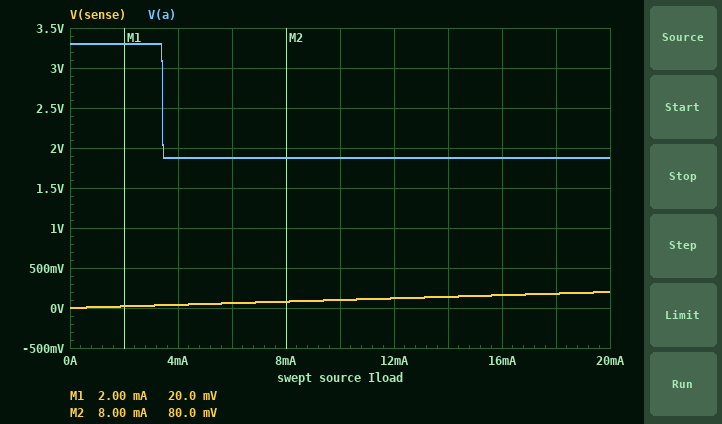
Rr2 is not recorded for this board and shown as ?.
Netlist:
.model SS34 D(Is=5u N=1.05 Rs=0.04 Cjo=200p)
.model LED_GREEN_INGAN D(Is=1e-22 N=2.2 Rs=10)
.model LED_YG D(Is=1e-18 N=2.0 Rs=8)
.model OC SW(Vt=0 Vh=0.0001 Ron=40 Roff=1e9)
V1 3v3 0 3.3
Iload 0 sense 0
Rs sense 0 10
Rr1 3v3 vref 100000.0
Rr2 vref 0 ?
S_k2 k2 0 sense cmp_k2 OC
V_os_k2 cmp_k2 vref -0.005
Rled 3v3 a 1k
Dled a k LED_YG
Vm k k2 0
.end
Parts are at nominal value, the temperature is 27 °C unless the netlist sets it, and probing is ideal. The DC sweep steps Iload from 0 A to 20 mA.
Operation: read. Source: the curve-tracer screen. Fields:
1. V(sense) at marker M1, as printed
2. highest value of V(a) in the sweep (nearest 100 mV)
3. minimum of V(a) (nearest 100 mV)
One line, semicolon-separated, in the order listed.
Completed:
20.0 mV; 3.3 V; 1.9 V
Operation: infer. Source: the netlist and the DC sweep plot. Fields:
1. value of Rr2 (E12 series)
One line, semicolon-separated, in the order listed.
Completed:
1.2 kΩ
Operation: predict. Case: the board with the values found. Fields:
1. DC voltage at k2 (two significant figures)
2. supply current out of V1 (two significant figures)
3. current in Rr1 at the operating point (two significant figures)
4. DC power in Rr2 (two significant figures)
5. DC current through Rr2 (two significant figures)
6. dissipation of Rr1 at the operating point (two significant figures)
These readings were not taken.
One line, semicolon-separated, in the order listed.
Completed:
2.2 V; 33 µA; 33 µA; 1.3 µW; 33 µA; 110 µW
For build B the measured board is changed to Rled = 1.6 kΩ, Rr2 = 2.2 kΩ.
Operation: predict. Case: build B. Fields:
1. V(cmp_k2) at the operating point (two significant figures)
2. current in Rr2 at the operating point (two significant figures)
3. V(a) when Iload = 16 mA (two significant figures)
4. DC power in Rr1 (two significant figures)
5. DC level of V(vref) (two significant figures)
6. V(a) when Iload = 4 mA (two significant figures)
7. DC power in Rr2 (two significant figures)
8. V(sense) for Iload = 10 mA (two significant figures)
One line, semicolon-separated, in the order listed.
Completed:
66 mV; 32 µA; 1.8 V; 100 µW; 71 mV; 3.3 V; 2.3 µW; 100 mV
